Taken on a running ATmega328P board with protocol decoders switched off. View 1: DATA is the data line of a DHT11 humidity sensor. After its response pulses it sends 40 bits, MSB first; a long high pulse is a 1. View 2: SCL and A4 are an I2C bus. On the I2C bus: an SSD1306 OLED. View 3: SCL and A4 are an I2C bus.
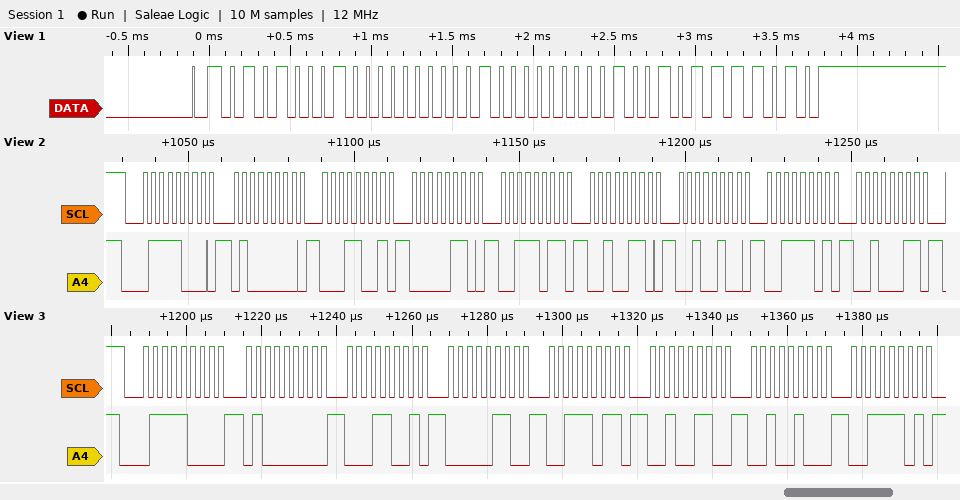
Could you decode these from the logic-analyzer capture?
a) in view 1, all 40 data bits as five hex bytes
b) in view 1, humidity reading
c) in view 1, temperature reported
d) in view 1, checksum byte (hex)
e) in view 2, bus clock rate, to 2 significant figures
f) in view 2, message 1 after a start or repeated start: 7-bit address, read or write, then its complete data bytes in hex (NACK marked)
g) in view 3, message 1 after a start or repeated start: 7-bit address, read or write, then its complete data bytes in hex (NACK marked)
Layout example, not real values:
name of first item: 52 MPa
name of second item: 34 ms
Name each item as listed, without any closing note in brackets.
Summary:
in view 1, all 40 data bits as five hex bytes: 51 00 20 09 7A
in view 1, humidity reading: 81 %
in view 1, temperature reported: 32.9 °C
in view 1, checksum byte: 0x7A
in view 2, bus clock rate, to 2 significant figures: 400 kHz
in view 2, message 1 after a start or repeated start: 7-bit address, read or write, then its complete data bytes in hex: 0x3C write: 40 19 06 3B 26 24 3D 23
in view 3, message 1 after a start or repeated start: 7-bit address, read or write, then its complete data bytes in hex: 0x3C write: 40 19 06 3B 26 24 3D
